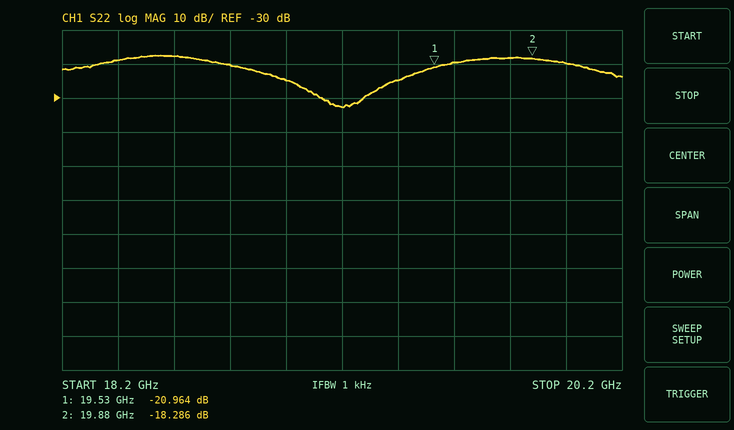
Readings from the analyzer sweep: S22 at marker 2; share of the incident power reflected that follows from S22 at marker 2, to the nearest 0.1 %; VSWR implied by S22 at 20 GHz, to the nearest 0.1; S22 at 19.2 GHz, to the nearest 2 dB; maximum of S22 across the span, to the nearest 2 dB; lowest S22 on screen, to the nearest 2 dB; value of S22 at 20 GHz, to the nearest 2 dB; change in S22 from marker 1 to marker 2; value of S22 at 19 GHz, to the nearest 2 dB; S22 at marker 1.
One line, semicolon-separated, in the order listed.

-18.286 dB; 1.5 %; 1.2; -32 dB; -18 dB; -32 dB; -20 dB; 2.678 dB; -24 dB; -20.964 dB
